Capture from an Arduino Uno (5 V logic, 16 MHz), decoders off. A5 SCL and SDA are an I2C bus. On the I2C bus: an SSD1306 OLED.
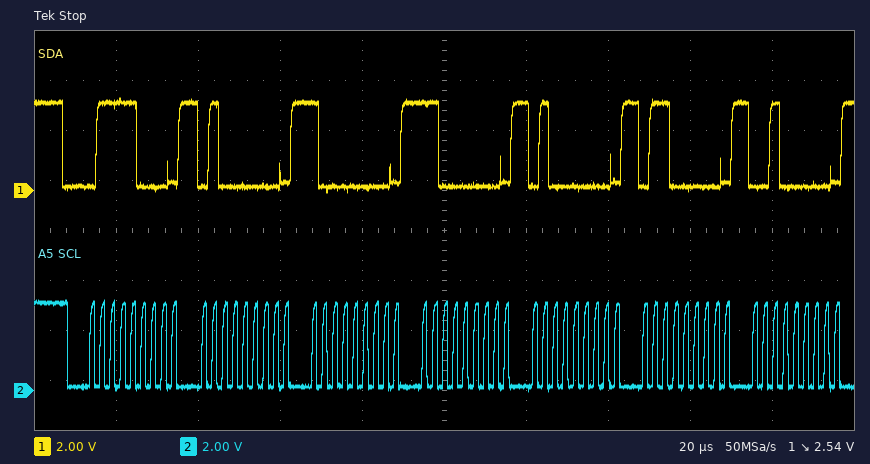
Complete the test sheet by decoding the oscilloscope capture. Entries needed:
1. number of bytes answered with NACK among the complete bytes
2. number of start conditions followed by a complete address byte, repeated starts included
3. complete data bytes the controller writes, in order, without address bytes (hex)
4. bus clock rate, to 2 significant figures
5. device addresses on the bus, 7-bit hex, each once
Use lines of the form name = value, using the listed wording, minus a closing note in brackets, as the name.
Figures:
number of bytes answered with NACK among the complete bytes = 0
number of start conditions followed by a complete address byte, repeated starts included = 1
complete data bytes the controller writes, in order, without address bytes = 40 80 C0 40 60 20
bus clock rate, to 2 significant figures = 400 kHz
device addresses on the bus, 7-bit hex, each once = 0x3C
